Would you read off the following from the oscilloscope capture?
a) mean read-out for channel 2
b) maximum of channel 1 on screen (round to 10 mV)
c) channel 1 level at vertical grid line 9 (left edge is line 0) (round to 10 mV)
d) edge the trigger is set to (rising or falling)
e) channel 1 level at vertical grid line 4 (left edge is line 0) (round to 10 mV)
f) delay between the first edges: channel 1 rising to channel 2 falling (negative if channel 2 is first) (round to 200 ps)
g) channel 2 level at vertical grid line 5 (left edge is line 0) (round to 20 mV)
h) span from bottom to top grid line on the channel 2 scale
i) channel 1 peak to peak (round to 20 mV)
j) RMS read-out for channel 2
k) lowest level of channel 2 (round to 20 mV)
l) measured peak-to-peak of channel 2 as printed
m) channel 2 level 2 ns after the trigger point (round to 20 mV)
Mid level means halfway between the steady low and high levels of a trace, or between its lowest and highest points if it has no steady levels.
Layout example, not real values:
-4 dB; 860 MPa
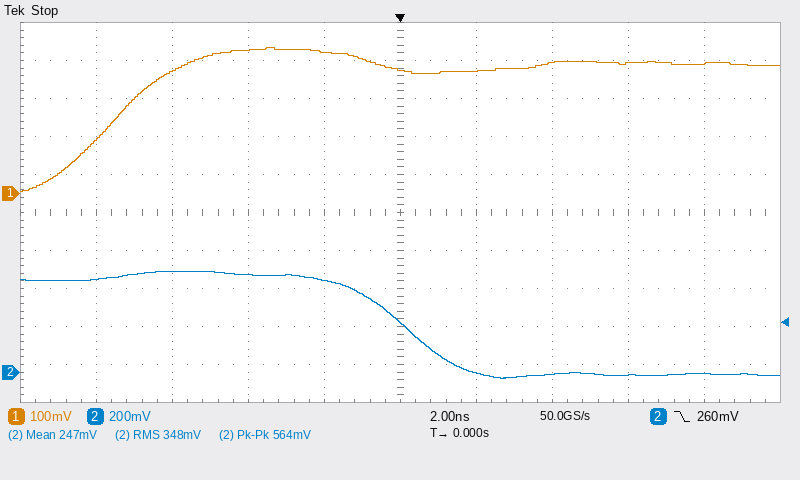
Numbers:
247 mV; 380 mV; 340 mV; falling; 370 mV; +7.6 ns; 260 mV; 2 V; 380 mV; 348 mV; -40 mV; 564 mV; 0 mV
